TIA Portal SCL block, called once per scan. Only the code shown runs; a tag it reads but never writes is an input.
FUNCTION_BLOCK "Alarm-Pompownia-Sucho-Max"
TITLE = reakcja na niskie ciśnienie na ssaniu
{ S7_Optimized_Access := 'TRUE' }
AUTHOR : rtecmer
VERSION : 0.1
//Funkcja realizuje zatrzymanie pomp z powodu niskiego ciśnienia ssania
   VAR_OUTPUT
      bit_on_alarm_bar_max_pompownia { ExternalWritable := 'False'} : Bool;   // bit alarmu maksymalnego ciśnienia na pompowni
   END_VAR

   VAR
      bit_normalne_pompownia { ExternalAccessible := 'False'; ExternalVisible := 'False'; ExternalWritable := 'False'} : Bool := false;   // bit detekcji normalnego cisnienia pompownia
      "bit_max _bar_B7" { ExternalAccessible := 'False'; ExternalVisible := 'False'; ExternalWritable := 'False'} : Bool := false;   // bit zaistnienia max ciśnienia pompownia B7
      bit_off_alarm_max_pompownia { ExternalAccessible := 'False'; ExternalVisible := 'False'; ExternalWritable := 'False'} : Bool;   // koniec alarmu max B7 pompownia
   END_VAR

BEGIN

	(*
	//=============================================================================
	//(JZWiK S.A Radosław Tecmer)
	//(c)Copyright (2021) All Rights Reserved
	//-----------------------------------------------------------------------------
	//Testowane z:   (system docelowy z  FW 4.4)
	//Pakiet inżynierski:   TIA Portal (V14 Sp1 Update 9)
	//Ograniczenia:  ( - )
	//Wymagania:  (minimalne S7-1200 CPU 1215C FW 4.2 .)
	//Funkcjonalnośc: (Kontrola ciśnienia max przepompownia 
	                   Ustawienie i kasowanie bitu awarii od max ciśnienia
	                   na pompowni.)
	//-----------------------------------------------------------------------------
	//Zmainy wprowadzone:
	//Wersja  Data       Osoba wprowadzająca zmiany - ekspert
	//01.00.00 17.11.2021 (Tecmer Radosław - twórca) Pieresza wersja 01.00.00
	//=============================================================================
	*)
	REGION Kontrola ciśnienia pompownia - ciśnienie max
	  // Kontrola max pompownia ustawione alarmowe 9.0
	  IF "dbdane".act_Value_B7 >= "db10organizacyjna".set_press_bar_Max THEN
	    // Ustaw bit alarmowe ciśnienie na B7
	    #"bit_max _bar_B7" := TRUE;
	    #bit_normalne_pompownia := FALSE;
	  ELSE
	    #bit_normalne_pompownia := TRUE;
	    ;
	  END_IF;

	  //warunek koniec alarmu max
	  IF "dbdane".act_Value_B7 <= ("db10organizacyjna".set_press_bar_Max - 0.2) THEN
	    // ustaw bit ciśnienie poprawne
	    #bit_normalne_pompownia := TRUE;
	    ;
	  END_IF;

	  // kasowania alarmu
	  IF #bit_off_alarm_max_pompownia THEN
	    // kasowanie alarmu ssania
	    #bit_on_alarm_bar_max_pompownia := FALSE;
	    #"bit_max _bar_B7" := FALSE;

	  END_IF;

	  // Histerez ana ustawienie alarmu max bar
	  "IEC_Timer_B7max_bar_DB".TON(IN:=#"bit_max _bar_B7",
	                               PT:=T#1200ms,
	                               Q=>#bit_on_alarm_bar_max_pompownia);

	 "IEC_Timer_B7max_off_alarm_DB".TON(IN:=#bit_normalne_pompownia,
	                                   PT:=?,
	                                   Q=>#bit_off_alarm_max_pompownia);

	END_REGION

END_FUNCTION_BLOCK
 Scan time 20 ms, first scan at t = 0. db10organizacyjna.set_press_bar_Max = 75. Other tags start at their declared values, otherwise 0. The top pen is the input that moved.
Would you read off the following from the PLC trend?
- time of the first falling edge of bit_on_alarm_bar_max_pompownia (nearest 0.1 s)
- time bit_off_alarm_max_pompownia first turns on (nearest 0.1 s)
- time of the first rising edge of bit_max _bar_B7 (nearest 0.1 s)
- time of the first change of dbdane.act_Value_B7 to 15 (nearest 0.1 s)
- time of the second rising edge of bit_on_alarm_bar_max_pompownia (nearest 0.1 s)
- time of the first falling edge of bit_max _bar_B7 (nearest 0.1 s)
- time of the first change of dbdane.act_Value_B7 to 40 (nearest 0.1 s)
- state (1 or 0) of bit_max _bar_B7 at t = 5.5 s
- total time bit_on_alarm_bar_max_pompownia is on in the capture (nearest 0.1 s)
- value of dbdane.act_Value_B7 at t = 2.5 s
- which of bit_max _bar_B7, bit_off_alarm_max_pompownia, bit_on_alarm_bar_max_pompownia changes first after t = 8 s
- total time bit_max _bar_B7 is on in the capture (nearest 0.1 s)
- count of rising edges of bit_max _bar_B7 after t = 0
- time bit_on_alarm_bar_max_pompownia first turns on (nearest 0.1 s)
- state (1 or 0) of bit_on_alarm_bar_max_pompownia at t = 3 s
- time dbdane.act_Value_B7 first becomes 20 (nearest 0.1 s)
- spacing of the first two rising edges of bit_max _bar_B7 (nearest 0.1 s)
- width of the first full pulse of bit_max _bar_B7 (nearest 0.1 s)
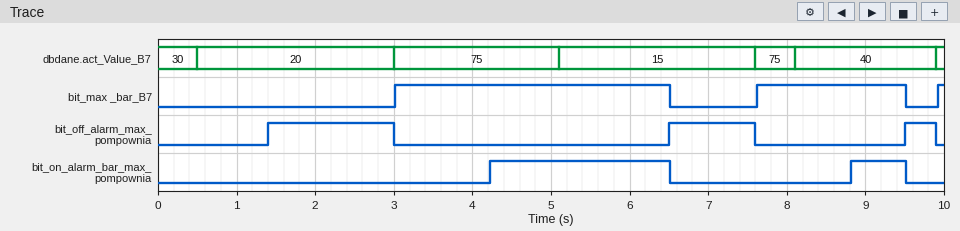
6.5 s
1.4 s
3.0 s
5.1 s
8.8 s
6.5 s
8.1 s
1
3.0 s
20
bit_on_alarm_bar_max_pompownia
5.5 s
3
4.2 s
0
0.5 s
4.6 s
3.5 s
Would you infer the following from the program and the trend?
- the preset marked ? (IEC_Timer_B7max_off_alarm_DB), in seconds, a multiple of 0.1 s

1.4 s
